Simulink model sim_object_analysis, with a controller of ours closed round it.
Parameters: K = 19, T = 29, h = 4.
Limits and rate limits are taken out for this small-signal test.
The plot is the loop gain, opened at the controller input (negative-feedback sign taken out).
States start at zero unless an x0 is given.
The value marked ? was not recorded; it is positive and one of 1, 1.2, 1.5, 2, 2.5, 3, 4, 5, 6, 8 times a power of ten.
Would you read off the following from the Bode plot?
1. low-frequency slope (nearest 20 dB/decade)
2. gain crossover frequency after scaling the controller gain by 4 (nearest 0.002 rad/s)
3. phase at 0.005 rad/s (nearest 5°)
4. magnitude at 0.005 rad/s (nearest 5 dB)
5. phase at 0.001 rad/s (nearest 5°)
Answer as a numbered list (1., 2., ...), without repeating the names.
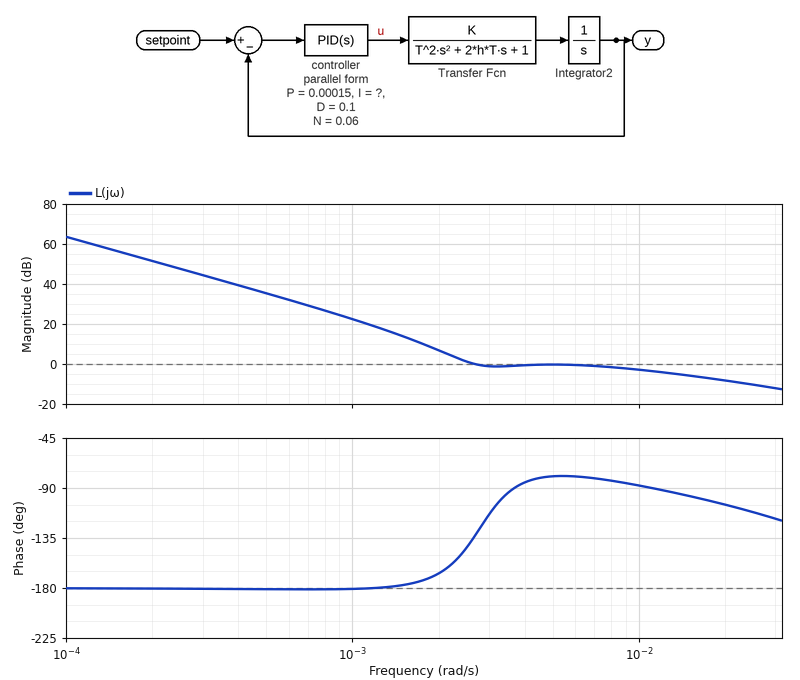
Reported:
1. -40 dB/decade
2. 0.030 rad/s
3. -80°
4. 0 dB
5. -180°
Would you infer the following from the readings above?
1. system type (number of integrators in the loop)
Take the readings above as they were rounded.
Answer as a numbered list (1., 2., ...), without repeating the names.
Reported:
1. 2
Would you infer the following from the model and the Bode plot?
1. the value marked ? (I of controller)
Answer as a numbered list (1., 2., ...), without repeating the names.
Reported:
1. 8e-07
